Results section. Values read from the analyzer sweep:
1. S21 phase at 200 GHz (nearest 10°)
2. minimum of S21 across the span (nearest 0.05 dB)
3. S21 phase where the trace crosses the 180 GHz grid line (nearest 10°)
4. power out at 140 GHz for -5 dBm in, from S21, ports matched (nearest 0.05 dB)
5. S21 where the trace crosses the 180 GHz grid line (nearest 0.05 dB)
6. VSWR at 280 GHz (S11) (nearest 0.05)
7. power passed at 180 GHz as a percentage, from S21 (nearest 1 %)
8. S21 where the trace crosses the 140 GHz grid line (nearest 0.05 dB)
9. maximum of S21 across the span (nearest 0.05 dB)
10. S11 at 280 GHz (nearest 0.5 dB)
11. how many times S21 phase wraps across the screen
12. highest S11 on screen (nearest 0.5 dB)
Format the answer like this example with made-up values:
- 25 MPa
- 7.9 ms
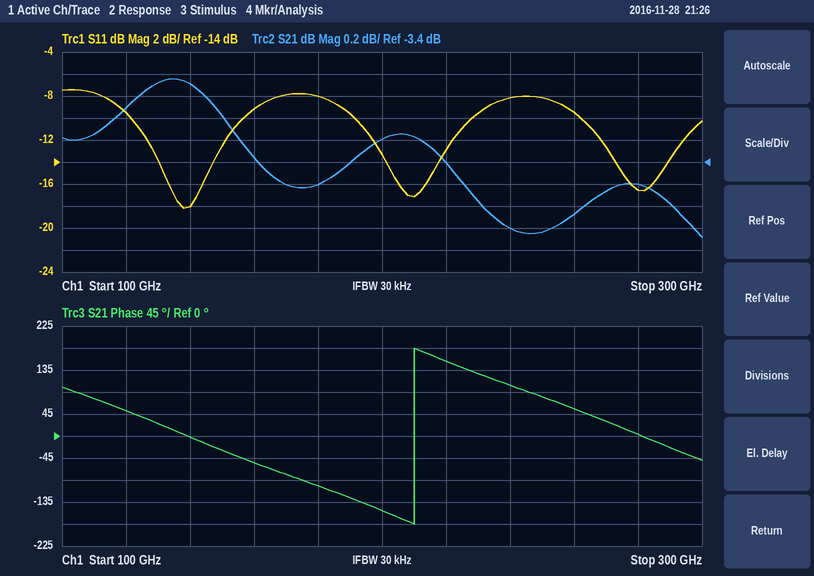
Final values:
- -150°
- -4.10 dB
- -100°
- -7.70 dBm
- -3.60 dB
- 1.35
- 44 %
- -2.70 dB
- -2.65 dB
- -16.5 dB
- 1
- -7.5 dB
